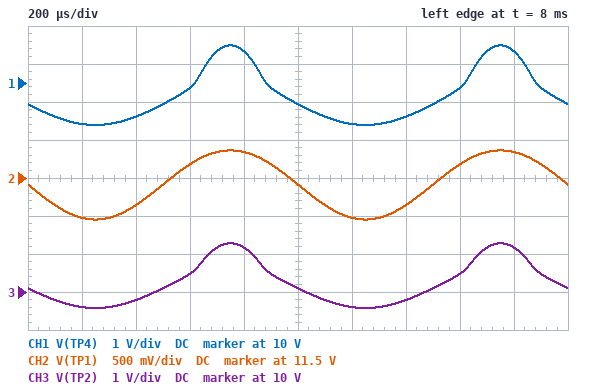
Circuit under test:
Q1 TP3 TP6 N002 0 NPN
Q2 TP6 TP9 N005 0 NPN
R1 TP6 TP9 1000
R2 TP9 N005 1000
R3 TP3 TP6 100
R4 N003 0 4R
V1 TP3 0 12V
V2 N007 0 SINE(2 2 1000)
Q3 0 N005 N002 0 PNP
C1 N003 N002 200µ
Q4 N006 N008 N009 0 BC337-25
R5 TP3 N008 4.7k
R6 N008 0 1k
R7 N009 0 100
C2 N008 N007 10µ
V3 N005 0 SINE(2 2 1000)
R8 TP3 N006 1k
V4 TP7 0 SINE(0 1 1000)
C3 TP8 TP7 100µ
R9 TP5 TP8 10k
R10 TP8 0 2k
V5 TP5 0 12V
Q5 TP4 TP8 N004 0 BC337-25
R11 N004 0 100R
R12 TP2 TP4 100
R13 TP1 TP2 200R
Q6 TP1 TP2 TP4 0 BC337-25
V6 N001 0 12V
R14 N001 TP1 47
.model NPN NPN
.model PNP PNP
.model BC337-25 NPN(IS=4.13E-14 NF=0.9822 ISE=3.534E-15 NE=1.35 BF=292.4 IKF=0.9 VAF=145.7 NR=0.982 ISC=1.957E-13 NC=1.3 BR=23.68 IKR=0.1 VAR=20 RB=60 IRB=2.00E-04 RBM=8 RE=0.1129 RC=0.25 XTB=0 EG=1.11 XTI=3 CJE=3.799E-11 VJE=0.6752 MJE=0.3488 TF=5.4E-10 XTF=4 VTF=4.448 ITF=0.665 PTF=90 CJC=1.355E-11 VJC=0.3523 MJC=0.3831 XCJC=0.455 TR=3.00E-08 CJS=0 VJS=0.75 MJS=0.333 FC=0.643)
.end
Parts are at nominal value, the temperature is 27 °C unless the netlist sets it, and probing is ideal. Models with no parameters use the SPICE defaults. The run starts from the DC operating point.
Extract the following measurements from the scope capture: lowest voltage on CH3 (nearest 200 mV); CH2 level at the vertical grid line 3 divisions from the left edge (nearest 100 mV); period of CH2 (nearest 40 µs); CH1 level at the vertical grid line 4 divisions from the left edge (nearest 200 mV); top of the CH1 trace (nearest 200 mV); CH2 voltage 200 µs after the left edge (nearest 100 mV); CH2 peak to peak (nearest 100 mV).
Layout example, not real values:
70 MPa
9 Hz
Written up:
9.6 V
11.7 V
1.00 ms
10.8 V
11.0 V
11.0 V
900 mV
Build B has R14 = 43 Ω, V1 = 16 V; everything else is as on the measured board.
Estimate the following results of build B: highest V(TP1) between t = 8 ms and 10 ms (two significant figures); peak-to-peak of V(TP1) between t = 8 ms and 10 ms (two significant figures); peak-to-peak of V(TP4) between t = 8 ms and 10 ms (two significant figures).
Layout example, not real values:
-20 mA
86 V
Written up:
12 V
830 mV
2.0 V
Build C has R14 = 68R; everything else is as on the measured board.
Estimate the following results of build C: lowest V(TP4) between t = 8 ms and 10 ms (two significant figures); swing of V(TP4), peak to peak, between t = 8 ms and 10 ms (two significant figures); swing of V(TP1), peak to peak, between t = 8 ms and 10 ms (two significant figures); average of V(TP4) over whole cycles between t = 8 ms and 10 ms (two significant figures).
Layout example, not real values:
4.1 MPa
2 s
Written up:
8.4 V
2.5 V
1.3 V
9.4 V
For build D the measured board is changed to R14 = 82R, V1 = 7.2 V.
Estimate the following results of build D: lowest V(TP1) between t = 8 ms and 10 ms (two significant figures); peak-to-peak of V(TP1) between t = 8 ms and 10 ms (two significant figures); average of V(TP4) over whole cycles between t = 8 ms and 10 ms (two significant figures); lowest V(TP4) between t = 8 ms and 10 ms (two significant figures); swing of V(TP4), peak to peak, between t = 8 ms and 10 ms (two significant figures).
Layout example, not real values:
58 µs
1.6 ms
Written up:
10 V
1.6 V
9.2 V
8.1 V
2.8 V
